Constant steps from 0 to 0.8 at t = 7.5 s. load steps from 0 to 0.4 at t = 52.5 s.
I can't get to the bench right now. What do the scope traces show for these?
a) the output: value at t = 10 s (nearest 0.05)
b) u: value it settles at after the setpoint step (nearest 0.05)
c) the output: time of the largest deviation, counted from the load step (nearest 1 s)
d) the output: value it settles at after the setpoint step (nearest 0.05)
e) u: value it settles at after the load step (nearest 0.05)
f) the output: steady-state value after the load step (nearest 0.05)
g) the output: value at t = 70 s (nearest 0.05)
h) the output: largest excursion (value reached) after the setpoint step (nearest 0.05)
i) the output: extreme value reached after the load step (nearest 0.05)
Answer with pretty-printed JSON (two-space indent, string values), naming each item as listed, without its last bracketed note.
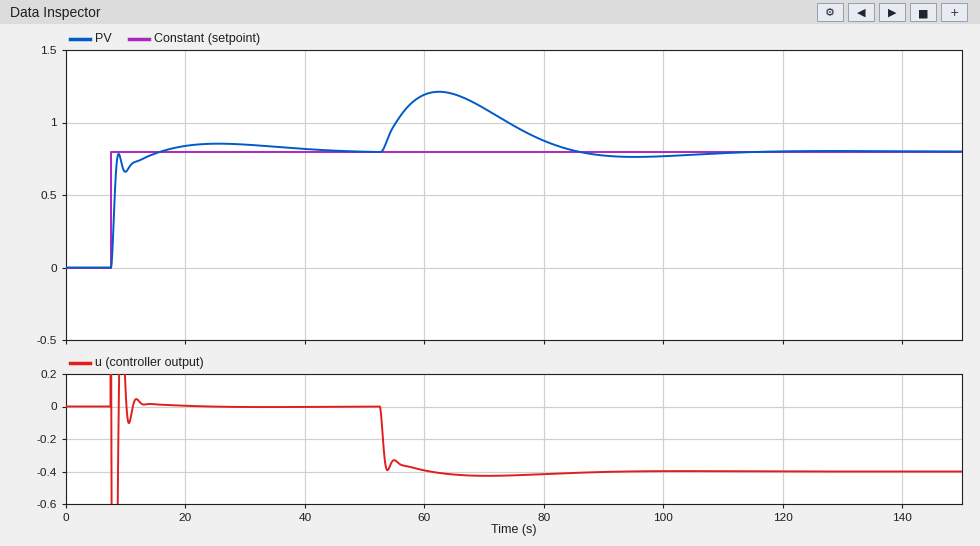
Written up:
{
  "the output: value at t = 10 s": "0.65",
  "u: value it settles at after the setpoint step": "0.00",
  "the output: time of the largest deviation, counted from the load step": "10 s",
  "the output: value it settles at after the setpoint step": "0.80",
  "u: value it settles at after the load step": "-0.40",
  "the output: steady-state value after the load step": "0.80",
  "the output: value at t = 70 s": "1.10",
  "the output: largest excursion (value reached) after the setpoint step": "0.85",
  "the output: extreme value reached after the load step": "1.20"
}
